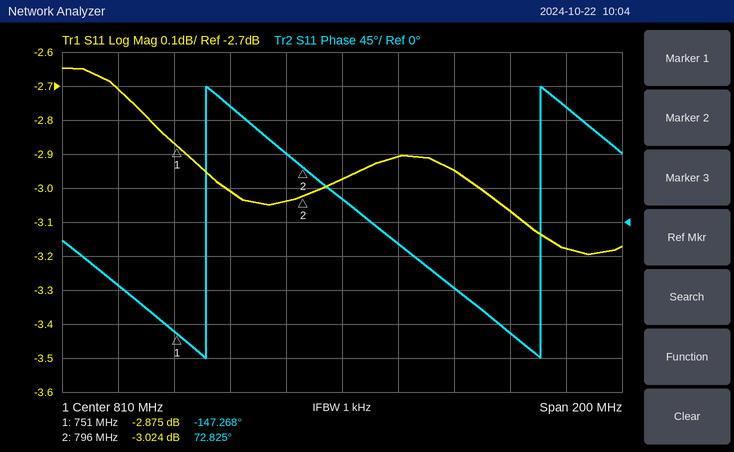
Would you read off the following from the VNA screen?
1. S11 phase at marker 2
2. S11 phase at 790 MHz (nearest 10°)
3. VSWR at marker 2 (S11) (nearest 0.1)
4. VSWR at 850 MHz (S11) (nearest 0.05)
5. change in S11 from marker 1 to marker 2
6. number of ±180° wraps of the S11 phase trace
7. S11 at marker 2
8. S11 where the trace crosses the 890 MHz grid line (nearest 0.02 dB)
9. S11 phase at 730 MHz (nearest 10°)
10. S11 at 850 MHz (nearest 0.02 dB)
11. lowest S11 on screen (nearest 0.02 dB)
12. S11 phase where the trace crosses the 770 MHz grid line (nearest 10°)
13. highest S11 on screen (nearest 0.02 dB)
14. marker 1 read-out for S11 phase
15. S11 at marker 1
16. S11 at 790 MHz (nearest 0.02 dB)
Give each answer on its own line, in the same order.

72.825°
90°
5.8
5.95
-0.149 dB
2
-3.024 dB
-3.18 dB
-80°
-2.94 dB
-3.20 dB
150°
-2.64 dB
-147.268°
-2.875 dB
-3.04 dB
